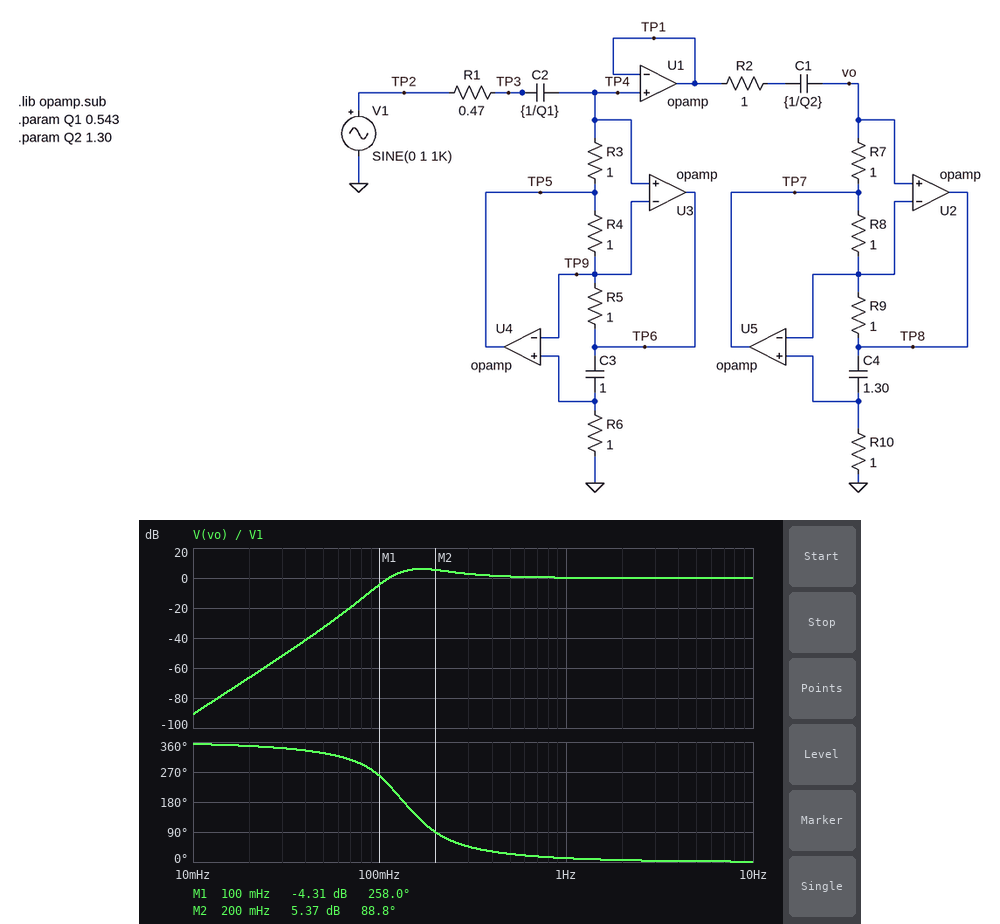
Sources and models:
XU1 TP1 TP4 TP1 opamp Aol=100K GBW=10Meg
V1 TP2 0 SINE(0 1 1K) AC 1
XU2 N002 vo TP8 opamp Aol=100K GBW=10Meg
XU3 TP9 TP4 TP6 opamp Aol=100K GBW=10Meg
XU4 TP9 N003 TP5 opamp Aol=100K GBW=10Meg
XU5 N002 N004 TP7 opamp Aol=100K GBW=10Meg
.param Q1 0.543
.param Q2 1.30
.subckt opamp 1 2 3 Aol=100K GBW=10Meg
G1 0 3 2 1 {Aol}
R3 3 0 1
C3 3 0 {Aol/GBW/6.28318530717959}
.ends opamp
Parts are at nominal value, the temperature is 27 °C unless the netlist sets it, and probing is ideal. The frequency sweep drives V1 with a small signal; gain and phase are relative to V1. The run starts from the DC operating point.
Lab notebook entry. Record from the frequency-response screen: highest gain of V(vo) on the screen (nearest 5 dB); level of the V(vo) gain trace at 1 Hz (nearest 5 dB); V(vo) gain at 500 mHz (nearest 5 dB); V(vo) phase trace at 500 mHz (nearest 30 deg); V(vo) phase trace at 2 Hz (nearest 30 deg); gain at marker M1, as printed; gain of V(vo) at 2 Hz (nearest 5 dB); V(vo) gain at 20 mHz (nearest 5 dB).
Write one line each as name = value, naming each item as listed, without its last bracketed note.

highest gain of V(vo) on the screen = 5 dB
level of the V(vo) gain trace at 1 Hz = 0 dB
V(vo) gain at 500 mHz = 0 dB
V(vo) phase trace at 500 mHz = 30 deg
V(vo) phase trace at 2 Hz = 0 deg
gain at marker M1, as printed = -4.31 dB
gain of V(vo) at 2 Hz = 0 dB
V(vo) gain at 20 mHz = -65 dB
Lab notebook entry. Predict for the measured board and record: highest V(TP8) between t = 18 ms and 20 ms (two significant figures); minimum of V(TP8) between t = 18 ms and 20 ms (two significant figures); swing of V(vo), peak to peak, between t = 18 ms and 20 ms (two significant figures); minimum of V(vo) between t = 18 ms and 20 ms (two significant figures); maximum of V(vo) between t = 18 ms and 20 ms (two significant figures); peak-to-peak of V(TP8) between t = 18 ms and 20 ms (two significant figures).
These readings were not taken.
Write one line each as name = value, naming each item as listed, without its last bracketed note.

highest V(TP8) between t = 18 ms and 20 ms = 1.0 V
minimum of V(TP8) between t = 18 ms and 20 ms = -1.0 V
swing of V(vo), peak to peak, between t = 18 ms and 20 ms = 2.0 V
minimum of V(vo) between t = 18 ms and 20 ms = -1.0 V
maximum of V(vo) between t = 18 ms and 20 ms = 1.0 V
peak-to-peak of V(TP8) between t = 18 ms and 20 ms = 2.0 V
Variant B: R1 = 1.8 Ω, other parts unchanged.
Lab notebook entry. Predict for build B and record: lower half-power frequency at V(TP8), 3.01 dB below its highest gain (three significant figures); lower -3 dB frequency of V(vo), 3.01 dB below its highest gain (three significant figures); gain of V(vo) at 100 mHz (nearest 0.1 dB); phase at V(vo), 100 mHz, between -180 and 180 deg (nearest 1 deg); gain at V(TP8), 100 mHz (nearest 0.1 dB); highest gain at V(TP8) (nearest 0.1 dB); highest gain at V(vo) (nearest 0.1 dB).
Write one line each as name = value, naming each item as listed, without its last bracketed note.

lower half-power frequency at V(TP8), 3.01 dB below its highest gain = 144 mHz
lower -3 dB frequency of V(vo), 3.01 dB below its highest gain = 160 mHz
gain of V(vo) at 100 mHz = -15.1 dB
phase at V(vo), 100 mHz, between -180 and 180 deg = -121 deg
gain at V(TP8), 100 mHz = -11.1 dB
highest gain at V(TP8) = 0.4 dB
highest gain at V(vo) = 0 dB
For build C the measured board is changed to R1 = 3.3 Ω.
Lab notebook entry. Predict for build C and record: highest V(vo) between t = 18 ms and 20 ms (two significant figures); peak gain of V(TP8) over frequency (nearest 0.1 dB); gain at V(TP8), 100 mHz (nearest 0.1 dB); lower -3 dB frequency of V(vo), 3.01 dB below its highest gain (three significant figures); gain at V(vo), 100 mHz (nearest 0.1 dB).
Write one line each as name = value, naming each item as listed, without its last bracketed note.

highest V(vo) between t = 18 ms and 20 ms = 1.0 V
peak gain of V(TP8) over frequency = 0 dB
gain at V(TP8), 100 mHz = -16.3 dB
lower -3 dB frequency of V(vo), 3.01 dB below its highest gain = 413 mHz
gain at V(vo), 100 mHz = -20.3 dB
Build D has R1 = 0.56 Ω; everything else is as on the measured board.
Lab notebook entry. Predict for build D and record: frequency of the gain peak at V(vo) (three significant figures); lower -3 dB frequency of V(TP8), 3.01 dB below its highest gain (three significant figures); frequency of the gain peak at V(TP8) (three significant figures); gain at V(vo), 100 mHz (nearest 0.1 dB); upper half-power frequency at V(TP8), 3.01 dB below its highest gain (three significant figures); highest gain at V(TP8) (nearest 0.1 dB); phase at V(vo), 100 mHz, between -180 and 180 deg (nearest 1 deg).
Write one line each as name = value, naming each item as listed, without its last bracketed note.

frequency of the gain peak at V(vo) = 174 mHz
lower -3 dB frequency of V(TP8), 3.01 dB below its highest gain = 123 mHz
frequency of the gain peak at V(TP8) = 165 mHz
gain at V(vo), 100 mHz = -5.6 dB
upper half-power frequency at V(TP8), 3.01 dB below its highest gain = 263 mHz
highest gain at V(TP8) = 7.2 dB
phase at V(vo), 100 mHz, between -180 and 180 deg = -106 deg
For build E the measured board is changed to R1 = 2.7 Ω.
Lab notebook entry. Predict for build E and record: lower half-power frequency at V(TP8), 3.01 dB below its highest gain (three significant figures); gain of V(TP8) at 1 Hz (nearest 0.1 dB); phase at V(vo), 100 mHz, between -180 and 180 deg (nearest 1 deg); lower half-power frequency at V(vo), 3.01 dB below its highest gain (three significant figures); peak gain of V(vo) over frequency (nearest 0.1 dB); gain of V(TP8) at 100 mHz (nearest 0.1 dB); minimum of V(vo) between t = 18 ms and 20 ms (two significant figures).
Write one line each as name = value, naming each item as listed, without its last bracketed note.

lower half-power frequency at V(TP8), 3.01 dB below its highest gain = 187 mHz
gain of V(TP8) at 1 Hz = -0.4 dB
phase at V(vo), 100 mHz, between -180 and 180 deg = -124 deg
lower half-power frequency at V(vo), 3.01 dB below its highest gain = 273 mHz
peak gain of V(vo) over frequency = 0 dB
gain of V(TP8) at 100 mHz = -14.6 dB
minimum of V(vo) between t = 18 ms and 20 ms = -1.0 V
